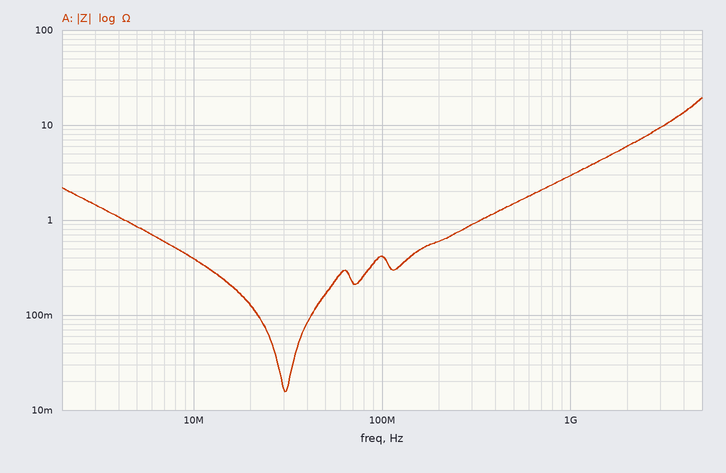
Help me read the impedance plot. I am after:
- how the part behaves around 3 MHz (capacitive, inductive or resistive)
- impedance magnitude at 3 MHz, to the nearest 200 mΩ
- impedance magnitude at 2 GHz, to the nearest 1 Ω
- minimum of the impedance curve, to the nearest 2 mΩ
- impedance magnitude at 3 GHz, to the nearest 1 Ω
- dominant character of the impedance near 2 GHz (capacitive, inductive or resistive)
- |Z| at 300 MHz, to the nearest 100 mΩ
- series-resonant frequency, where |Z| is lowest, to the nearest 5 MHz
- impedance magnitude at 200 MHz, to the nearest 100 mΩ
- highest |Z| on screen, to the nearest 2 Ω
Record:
capacitive
1.4 Ω
6 Ω
16 mΩ
9 Ω
inductive
900 mΩ
30 MHz
600 mΩ
20 Ω
